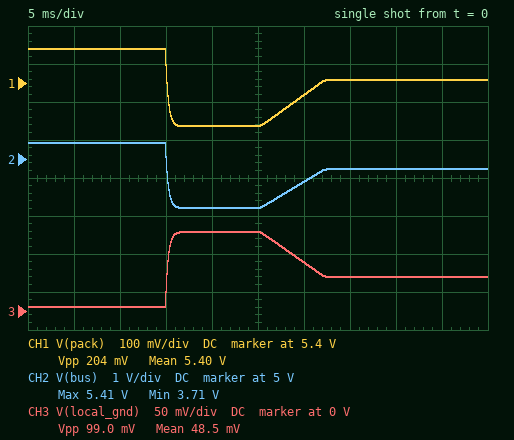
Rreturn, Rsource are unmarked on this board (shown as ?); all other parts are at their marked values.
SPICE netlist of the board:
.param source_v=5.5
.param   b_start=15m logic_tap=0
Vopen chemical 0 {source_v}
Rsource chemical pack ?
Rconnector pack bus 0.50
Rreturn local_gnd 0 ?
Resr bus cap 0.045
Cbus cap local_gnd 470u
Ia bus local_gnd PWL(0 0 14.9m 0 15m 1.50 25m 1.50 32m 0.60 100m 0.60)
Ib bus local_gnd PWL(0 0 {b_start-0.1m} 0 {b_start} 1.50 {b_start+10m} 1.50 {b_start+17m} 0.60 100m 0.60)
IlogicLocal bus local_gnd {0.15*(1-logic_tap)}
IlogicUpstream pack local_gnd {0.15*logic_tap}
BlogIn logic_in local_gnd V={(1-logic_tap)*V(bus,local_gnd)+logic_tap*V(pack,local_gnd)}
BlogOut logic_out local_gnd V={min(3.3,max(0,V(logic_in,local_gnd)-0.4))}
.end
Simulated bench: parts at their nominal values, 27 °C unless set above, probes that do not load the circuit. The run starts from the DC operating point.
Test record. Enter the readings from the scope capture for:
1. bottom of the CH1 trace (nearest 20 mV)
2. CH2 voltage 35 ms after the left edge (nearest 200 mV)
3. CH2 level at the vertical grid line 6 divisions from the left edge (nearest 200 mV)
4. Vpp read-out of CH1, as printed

5.28 V
4.8 V
4.4 V
204 mV
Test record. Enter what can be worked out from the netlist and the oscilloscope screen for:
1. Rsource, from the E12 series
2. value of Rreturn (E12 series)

0.068 Ω
0.033 Ω
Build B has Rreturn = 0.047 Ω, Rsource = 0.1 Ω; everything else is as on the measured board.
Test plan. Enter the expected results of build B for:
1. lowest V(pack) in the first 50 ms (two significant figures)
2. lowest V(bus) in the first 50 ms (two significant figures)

5.2 V
3.6 V
